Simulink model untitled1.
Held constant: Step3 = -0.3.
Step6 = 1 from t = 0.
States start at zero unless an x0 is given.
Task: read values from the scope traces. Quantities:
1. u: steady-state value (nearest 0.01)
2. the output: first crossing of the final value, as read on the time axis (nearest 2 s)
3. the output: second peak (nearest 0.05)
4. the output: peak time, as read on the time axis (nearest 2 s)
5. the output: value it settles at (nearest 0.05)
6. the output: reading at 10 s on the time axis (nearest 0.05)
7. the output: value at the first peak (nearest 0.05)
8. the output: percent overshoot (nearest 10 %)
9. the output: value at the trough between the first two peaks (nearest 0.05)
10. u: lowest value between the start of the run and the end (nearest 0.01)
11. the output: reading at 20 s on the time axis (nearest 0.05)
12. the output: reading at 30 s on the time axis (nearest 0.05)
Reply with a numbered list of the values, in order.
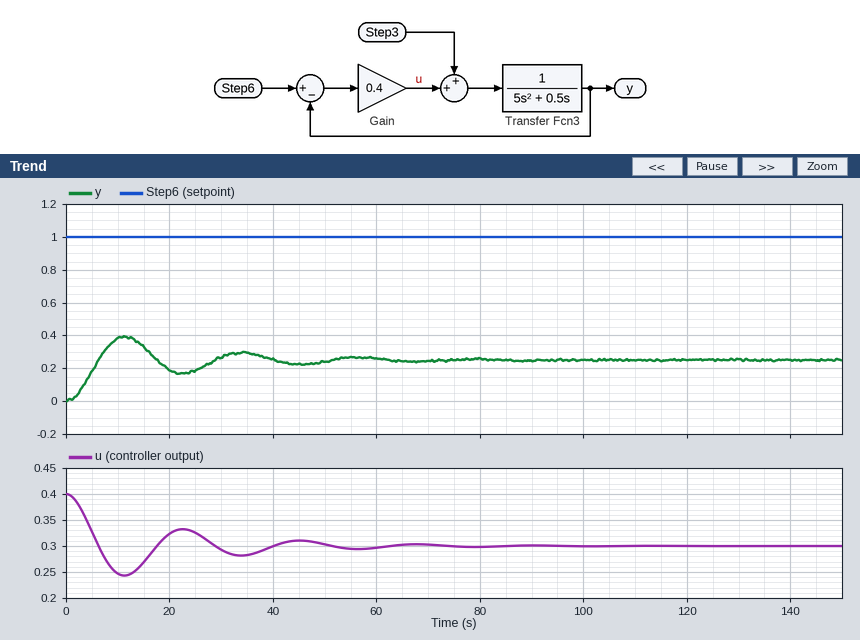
1. 0.30
2. 6 s
3. 0.30
4. 12 s
5. 0.25
6. 0.40
7. 0.40
8. 60 %
9. 0.15
10. 0.24
11. 0.20
12. 0.25
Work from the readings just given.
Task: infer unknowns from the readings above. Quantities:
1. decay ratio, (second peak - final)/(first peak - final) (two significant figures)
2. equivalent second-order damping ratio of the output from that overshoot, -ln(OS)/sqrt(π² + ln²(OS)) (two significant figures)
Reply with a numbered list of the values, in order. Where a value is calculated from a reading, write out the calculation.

1. (0.3 - 0.25) / (0.4 - 0.25) = 0.33
2. ln(0.6) = -0.511; 0.511 / sqrt(9.870 + 0.261) = 0.16
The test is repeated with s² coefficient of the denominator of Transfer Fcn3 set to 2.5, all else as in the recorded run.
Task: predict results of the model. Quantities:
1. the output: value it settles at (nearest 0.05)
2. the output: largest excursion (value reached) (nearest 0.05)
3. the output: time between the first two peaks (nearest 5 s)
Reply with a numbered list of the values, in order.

1. 0.25
2. 0.35
3. 15 s
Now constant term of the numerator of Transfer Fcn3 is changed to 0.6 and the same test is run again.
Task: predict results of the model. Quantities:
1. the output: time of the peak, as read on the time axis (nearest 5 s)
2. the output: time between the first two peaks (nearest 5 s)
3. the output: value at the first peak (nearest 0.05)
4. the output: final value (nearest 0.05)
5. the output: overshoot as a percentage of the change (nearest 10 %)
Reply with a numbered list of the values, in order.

1. 15 s
2. 30 s
3. 0.35
4. 0.25
5. 50 %
